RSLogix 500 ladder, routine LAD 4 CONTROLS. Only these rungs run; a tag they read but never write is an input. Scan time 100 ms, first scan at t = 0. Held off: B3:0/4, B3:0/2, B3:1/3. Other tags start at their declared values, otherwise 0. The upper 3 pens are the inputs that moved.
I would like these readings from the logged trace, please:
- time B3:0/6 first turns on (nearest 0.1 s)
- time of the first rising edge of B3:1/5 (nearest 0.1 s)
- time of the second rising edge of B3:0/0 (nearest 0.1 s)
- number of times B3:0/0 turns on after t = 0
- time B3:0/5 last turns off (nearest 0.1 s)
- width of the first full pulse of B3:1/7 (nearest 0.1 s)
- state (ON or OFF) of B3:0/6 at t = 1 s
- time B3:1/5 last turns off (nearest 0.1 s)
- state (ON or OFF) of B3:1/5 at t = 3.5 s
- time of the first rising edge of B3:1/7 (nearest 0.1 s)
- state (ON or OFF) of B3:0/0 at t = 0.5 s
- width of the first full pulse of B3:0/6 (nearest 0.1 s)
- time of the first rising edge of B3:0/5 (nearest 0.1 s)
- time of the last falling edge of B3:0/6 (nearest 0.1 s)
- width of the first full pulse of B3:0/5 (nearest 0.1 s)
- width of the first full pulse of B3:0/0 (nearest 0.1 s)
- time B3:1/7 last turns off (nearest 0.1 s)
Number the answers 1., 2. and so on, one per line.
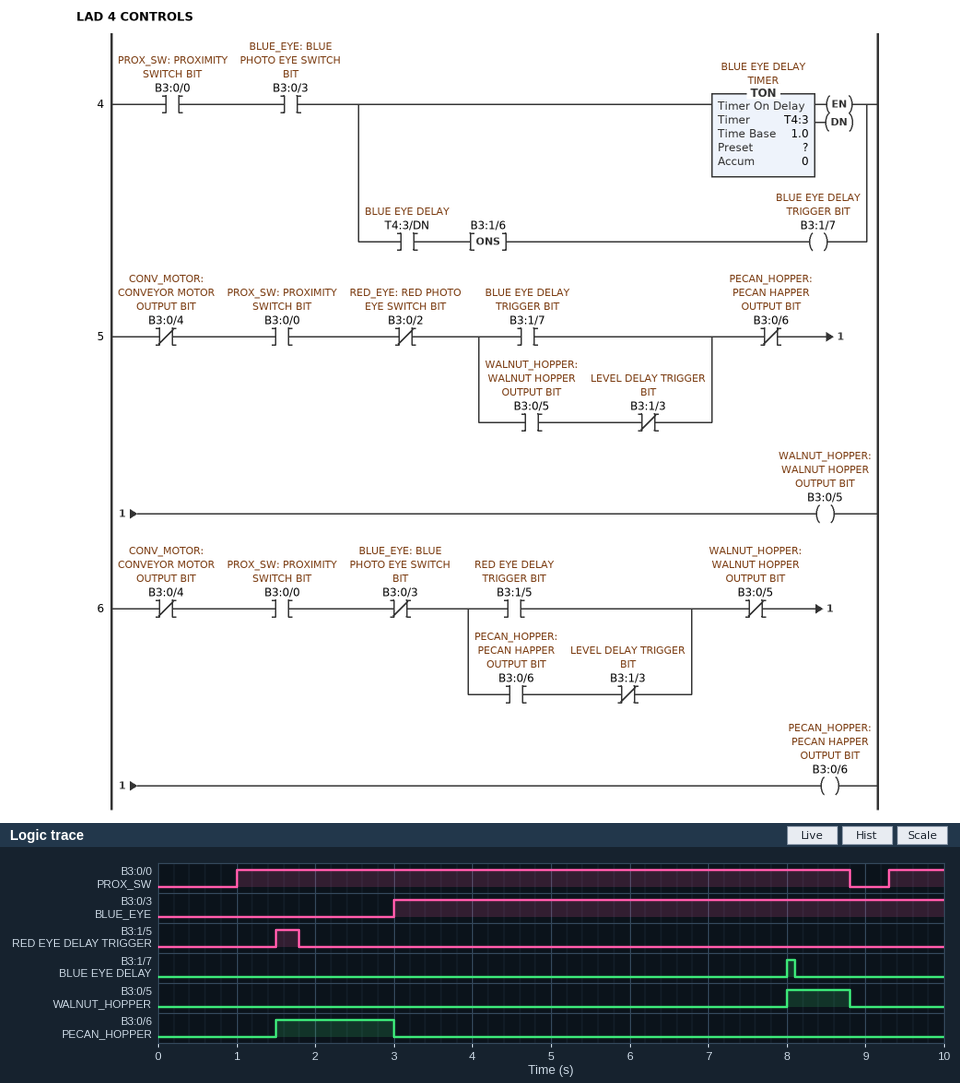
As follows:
1. 1.5 s
2. 1.5 s
3. 9.3 s
4. 2
5. 8.8 s
6. 0.1 s
7. OFF
8. 1.8 s
9. OFF
10. 8.0 s
11. OFF
12. 1.5 s
13. 8.0 s
14. 3.0 s
15. 0.8 s
16. 7.8 s
17. 8.1 s
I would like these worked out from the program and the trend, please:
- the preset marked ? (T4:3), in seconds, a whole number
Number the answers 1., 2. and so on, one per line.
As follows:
1. 5 s
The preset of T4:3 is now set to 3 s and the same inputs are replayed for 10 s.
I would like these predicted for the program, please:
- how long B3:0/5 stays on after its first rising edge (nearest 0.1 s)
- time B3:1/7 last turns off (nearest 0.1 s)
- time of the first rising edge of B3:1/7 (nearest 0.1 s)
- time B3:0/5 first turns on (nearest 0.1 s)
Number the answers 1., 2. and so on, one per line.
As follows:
1. 2.8 s
2. 6.1 s
3. 6.0 s
4. 6.0 s
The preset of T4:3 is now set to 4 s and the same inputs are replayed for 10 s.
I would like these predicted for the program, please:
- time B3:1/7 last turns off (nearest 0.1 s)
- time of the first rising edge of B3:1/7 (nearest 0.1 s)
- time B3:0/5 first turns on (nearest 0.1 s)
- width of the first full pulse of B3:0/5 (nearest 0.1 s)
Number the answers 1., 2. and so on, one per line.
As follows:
1. 7.1 s
2. 7.0 s
3. 7.0 s
4. 1.8 s
